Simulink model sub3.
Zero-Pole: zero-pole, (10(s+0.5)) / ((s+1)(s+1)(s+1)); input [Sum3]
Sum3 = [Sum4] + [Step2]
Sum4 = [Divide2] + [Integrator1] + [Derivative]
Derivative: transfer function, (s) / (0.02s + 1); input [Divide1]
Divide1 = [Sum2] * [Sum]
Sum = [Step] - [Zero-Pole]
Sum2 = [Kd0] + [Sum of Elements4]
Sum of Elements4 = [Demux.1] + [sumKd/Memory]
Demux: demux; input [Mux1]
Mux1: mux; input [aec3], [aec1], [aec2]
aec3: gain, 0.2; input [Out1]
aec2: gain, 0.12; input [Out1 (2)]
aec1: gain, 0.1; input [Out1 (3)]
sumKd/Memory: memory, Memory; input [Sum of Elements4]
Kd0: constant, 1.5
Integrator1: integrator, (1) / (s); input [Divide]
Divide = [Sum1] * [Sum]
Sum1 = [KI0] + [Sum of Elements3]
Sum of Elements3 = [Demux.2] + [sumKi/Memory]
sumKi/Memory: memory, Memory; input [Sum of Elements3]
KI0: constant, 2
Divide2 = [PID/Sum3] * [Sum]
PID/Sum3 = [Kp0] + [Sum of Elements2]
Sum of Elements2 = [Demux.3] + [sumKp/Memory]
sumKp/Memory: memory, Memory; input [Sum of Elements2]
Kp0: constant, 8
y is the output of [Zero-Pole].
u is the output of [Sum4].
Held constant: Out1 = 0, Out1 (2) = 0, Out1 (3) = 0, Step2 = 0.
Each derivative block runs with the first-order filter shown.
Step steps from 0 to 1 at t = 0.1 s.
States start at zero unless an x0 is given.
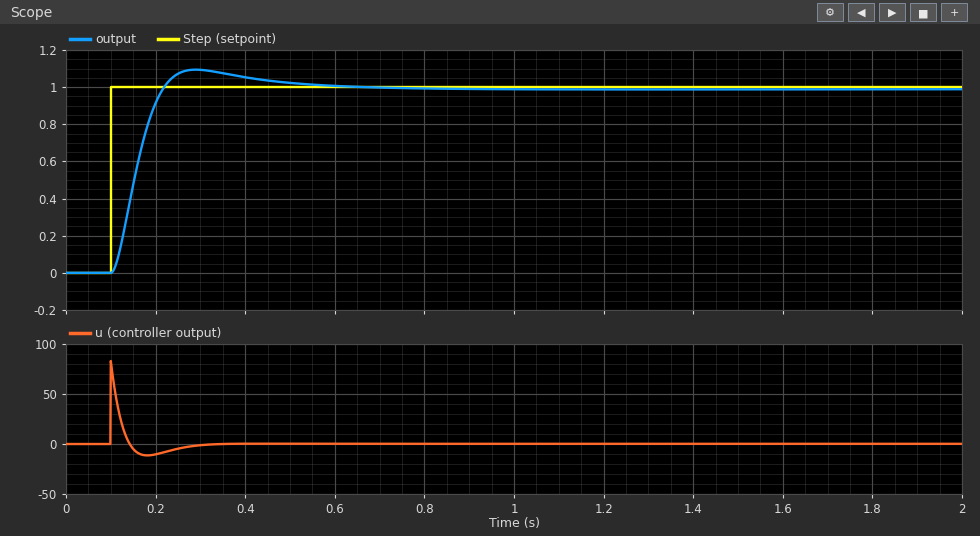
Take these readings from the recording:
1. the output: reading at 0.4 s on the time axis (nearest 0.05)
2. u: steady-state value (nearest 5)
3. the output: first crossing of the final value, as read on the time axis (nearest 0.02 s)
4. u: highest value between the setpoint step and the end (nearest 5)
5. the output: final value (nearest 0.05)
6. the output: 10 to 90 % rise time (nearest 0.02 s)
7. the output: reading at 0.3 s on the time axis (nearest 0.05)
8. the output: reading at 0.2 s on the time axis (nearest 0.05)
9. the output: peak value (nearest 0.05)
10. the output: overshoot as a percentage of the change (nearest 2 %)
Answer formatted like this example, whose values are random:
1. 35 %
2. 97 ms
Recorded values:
1. 1.05
2. 0
3. 0.22 s
4. 85
5. 1.00
6. 0.08 s
7. 1.10
8. 0.90
9. 1.10
10. 10 %
